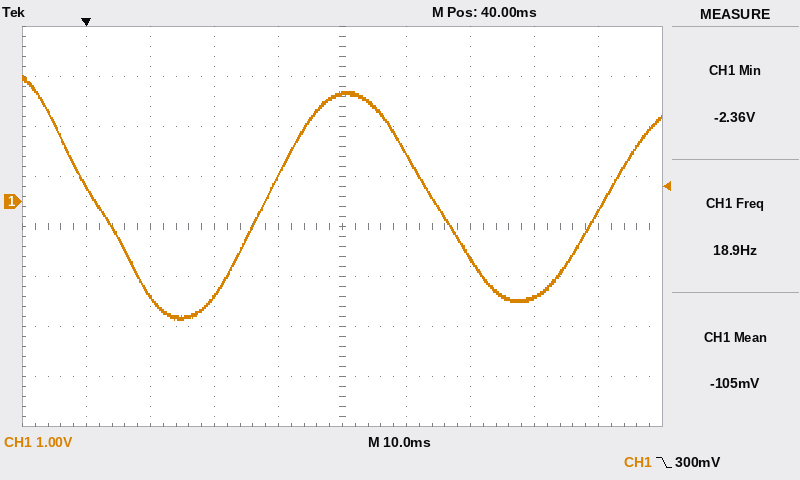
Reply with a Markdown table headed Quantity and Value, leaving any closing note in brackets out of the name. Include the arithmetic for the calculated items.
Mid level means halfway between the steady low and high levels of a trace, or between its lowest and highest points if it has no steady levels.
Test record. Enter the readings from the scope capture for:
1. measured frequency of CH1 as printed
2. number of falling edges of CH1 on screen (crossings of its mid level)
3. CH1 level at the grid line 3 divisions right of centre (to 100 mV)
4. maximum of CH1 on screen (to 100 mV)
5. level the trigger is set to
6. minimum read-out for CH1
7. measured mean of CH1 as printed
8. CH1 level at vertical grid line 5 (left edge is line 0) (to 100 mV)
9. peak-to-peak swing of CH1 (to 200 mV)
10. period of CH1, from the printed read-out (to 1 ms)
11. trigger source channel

| Quantity | Value |
|---|---|
| measured frequency of CH1 as printed | 18.9 Hz |
| number of falling edges of CH1 on screen | 2 |
| CH1 level at the grid line 3 divisions right of centre | -1.9 V |
| maximum of CH1 on screen | 2.5 V |
| level the trigger is set to | 300 mV |
| minimum read-out for CH1 | -2.36 V |
| measured mean of CH1 as printed | -105 mV |
| CH1 level at vertical grid line 5 (left edge is line 0) | 2.2 V |
| peak-to-peak swing of CH1 | 4.8 V |
| period of CH1, from the printed read-out | 1 / 18.9 Hz ≈ 53 ms |
| trigger source channel | CH1 |
